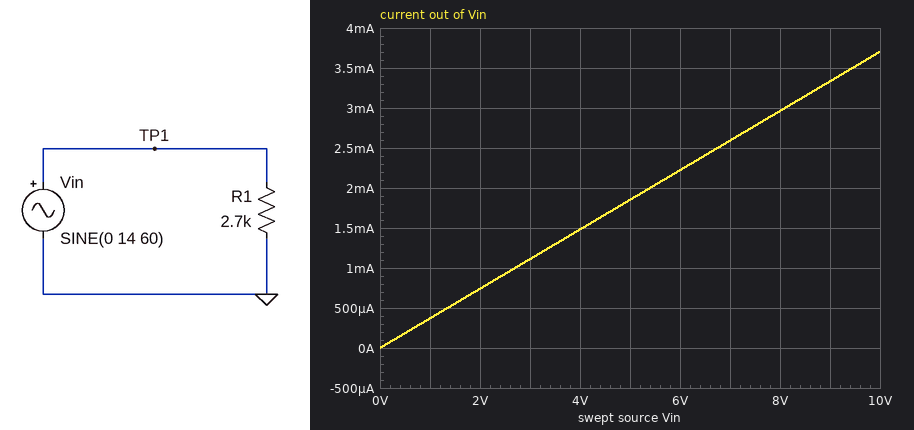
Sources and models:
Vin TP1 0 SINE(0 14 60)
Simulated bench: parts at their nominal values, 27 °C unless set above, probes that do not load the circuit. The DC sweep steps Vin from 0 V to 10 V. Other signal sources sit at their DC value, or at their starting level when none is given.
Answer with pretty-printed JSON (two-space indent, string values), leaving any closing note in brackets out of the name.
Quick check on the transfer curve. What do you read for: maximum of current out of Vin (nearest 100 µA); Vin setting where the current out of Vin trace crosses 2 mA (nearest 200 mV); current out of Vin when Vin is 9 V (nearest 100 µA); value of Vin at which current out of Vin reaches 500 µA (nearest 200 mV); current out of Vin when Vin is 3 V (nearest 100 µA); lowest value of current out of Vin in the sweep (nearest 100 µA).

{
  "maximum of current out of Vin": "3.7 mA",
  "Vin setting where the current out of Vin trace crosses 2 mA": "5.4 V",
  "current out of Vin when Vin is 9 V": "3.3 mA",
  "value of Vin at which current out of Vin reaches 500 µA": "1.4 V",
  "current out of Vin when Vin is 3 V": "1.1 mA",
  "lowest value of current out of Vin in the sweep": "0 A"
}
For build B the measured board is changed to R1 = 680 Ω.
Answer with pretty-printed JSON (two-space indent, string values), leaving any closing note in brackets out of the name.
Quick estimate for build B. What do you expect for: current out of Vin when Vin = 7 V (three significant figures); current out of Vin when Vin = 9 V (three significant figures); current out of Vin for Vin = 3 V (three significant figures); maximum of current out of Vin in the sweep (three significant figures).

{
  "current out of Vin when Vin = 7 V": "10.3 mA",
  "current out of Vin when Vin = 9 V": "13.2 mA",
  "current out of Vin for Vin = 3 V": "4.41 mA",
  "maximum of current out of Vin in the sweep": "14.7 mA"
}
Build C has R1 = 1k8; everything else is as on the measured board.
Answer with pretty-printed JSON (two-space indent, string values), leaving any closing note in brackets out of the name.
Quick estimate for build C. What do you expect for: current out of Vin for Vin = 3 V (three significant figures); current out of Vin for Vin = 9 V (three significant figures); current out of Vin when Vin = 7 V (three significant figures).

{
  "current out of Vin for Vin = 3 V": "1.67 mA",
  "current out of Vin for Vin = 9 V": "5.00 mA",
  "current out of Vin when Vin = 7 V": "3.89 mA"
}
